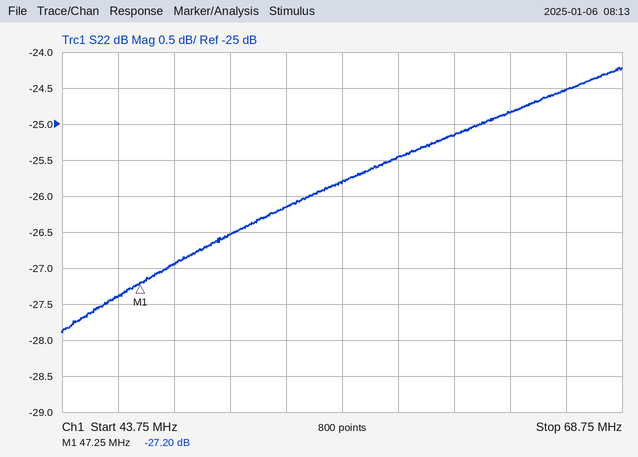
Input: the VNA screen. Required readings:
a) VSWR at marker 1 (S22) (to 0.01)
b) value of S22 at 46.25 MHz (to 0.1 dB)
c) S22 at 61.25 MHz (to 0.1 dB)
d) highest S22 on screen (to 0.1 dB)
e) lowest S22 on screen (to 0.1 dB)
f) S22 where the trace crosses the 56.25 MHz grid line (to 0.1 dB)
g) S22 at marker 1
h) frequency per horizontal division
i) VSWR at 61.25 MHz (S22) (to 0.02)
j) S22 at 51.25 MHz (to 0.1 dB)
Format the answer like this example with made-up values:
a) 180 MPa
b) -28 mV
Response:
a) 1.09
b) -27.4 dB
c) -25.2 dB
d) -24.2 dB
e) -27.9 dB
f) -25.8 dB
g) -27.20 dB
h) 2.5 MHz
i) 1.12
j) -26.5 dB
